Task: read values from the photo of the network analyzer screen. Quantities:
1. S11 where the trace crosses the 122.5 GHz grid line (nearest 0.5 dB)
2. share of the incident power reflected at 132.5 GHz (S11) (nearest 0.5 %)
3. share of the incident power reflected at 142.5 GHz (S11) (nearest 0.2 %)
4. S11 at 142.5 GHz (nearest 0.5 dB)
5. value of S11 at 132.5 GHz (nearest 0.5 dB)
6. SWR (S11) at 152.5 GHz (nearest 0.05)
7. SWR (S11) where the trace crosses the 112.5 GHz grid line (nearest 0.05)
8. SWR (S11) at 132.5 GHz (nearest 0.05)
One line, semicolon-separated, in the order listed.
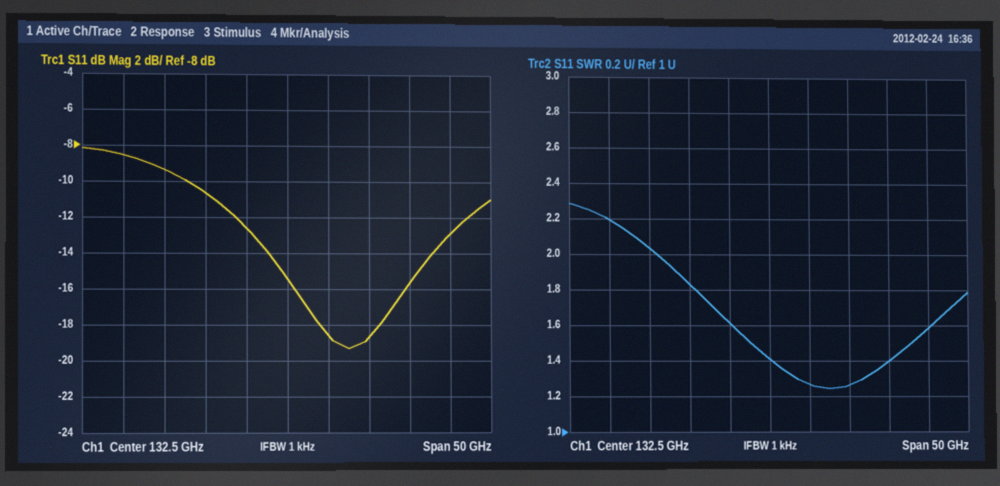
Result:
-10.5 dB; 3.0 %; 1.4 %; -18.5 dB; -15.5 dB; 1.60; 2.20; 1.40
